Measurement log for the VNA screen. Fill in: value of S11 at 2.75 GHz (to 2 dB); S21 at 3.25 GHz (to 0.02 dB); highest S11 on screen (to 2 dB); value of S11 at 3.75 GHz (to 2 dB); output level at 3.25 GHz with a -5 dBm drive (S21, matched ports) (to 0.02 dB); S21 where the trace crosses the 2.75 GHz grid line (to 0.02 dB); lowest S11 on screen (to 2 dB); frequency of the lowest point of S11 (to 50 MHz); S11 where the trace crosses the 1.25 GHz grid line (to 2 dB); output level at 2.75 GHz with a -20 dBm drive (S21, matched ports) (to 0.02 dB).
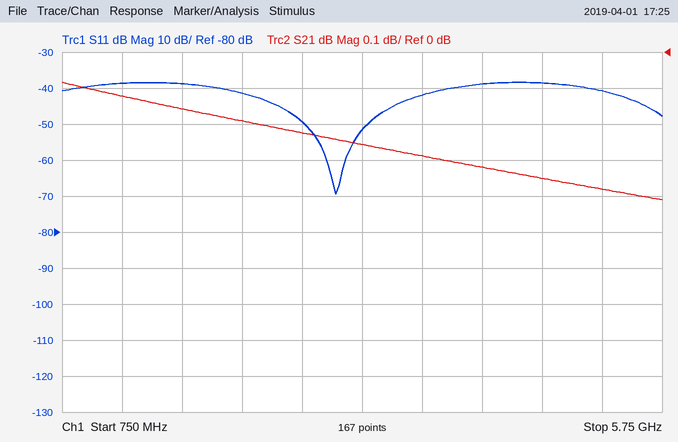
-50 dB
-0.26 dB
-38 dB
-42 dB
-5.26 dBm
-0.22 dB
-70 dB
3.05 GHz
-38 dB
-20.22 dBm
